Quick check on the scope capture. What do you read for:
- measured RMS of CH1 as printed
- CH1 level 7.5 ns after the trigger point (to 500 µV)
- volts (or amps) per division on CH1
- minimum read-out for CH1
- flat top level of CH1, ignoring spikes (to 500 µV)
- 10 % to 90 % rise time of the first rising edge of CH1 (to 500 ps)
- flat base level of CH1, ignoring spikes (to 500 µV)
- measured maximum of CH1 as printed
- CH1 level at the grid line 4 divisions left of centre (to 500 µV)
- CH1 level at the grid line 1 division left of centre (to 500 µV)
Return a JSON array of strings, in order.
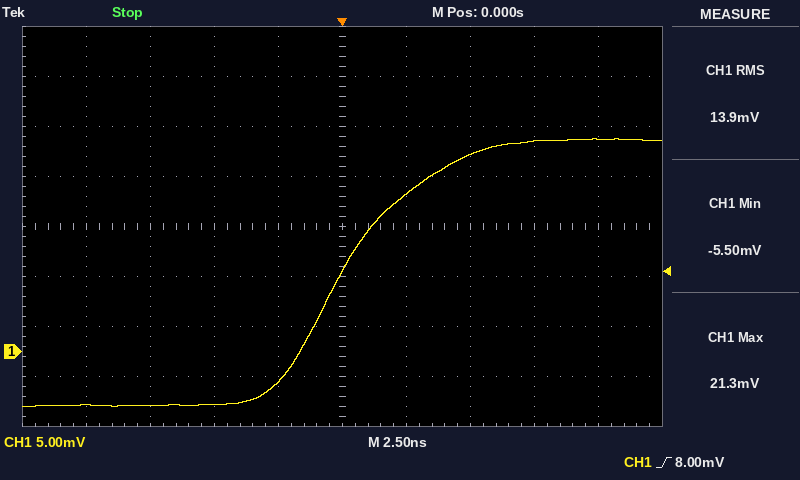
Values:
["13.9 mV", "21.0 mV", "5 mV", "-5.50 mV", "21.0 mV", "6.5 ns", "-5.5 mV", "21.3 mV", "-5.5 mV", "-3.0 mV"]
